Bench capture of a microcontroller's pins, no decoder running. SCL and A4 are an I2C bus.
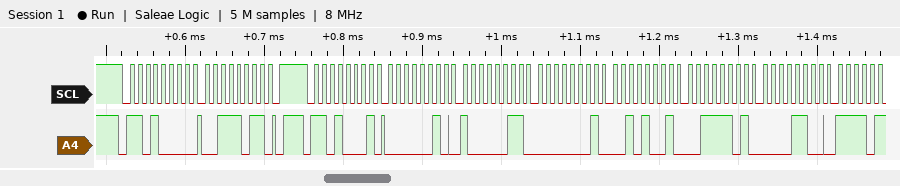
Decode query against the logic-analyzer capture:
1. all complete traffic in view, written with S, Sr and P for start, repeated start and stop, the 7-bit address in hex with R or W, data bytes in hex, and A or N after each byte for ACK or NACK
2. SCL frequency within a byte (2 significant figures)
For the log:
S 68W A 3B A P S 68R A 02 A 83 A 01 A 29 A 3D A 0C A
100 kHz
